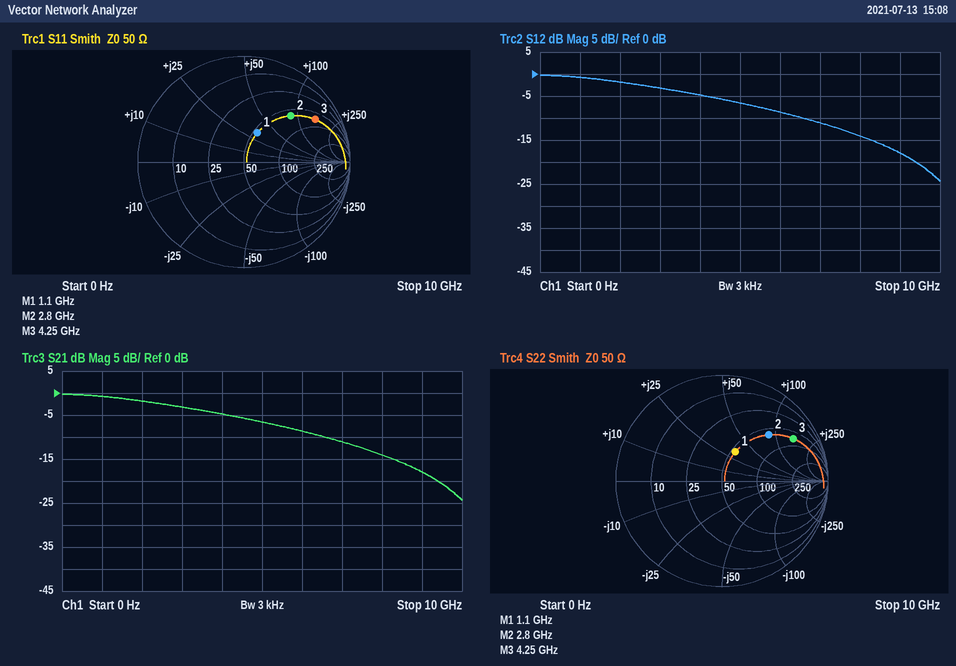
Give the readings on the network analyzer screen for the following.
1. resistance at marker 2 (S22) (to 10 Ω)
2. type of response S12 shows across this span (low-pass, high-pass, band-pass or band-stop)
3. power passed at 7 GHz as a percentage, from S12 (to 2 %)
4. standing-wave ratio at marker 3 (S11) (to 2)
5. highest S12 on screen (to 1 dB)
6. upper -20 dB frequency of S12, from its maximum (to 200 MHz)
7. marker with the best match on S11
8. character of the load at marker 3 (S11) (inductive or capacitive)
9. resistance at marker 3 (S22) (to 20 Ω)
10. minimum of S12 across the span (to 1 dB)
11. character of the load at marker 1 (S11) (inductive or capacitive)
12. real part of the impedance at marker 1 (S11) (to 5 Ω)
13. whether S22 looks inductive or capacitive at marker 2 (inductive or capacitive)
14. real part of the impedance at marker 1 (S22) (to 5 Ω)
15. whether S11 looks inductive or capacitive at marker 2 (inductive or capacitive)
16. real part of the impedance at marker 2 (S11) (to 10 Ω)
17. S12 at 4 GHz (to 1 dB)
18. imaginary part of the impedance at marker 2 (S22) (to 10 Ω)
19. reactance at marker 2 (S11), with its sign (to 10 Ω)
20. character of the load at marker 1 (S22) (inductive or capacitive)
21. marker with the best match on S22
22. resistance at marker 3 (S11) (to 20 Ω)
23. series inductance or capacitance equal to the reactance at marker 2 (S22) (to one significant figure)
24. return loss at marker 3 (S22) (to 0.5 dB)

60 Ω
low-pass
8 %
8
0 dB
9.4 GHz
marker 1
inductive
80 Ω
-24 dB
inductive
55 Ω
inductive
55 Ω
inductive
60 Ω
-5 dB
+90 Ω
+90 Ω
inductive
marker 1
80 Ω
5 nH
2.0 dB
